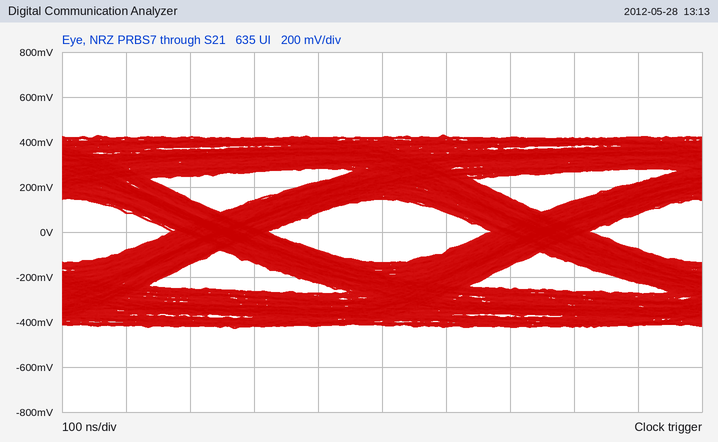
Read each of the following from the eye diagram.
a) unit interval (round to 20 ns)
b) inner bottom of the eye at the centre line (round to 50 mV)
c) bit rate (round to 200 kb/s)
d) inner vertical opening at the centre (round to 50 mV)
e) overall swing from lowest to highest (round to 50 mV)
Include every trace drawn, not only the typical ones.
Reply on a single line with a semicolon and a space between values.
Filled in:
500 ns; -150 mV; 2.0 Mb/s; 300 mV; 850 mV
